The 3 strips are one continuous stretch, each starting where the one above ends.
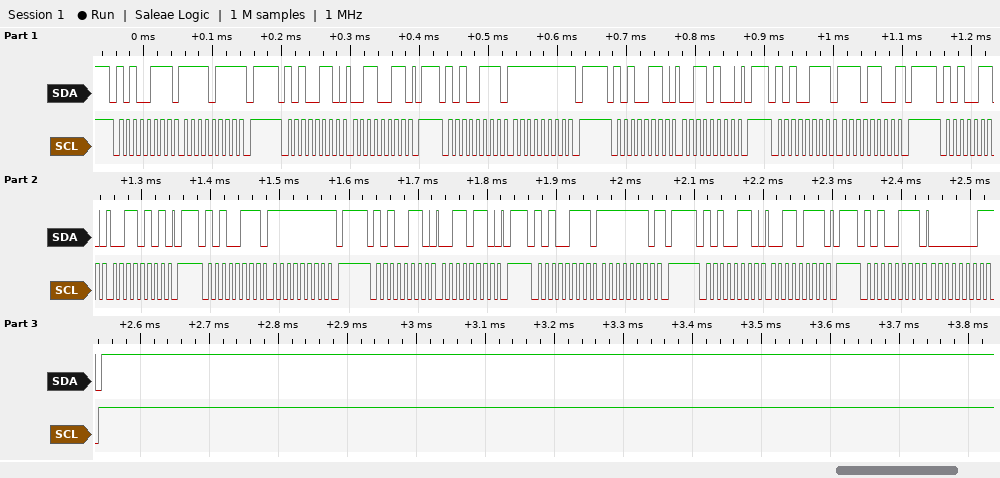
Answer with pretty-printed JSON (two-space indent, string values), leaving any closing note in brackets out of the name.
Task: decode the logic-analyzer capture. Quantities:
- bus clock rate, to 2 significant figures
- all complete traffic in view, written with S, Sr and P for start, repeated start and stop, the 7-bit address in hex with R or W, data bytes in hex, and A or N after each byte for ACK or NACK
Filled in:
{
  "bus clock rate, to 2 significant figures": "100 kHz",
  "all complete traffic in view, written with S, Sr and P for start, repeated start and stop, the 7-bit address in hex with R or W, data bytes in hex, and A or N after each byte for ACK or NACK": "S 53R A F7 N P S 53W A 33 A P S 53R A FF N P S 53W A 34 A P S 53R A EC N P S 53W A 35 A P S 53R A FF N P S 53W A 36 A P S 53R A FE N P S 53W A 37 A P S 53R A 01 N P"
}
